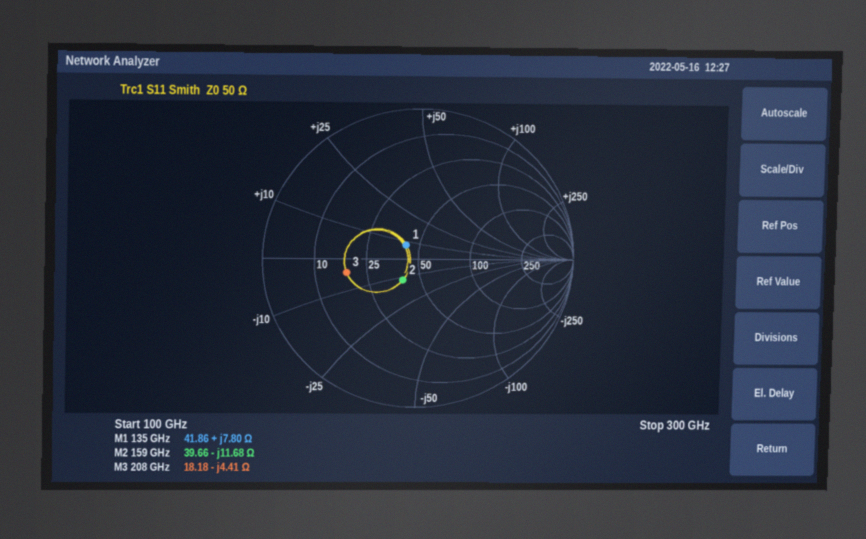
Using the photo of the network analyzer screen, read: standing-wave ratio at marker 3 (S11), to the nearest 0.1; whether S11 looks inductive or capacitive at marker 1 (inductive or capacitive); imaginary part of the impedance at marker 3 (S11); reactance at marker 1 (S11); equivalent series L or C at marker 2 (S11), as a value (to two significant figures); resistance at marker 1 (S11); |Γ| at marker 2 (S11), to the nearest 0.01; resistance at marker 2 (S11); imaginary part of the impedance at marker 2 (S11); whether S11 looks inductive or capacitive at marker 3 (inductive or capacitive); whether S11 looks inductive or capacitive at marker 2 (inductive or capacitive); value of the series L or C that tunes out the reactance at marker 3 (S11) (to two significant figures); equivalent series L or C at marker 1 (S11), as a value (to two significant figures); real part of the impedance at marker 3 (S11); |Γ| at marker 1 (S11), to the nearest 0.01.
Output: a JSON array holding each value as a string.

["2.8", "inductive", "-4.41 Ω", "+7.80 Ω", "86 fF", "41.86 Ω", "0.17", "39.66 Ω", "-11.68 Ω", "capacitive", "capacitive", "3.4 pH", "9.2 pH", "18.18 Ω", "0.12"]
